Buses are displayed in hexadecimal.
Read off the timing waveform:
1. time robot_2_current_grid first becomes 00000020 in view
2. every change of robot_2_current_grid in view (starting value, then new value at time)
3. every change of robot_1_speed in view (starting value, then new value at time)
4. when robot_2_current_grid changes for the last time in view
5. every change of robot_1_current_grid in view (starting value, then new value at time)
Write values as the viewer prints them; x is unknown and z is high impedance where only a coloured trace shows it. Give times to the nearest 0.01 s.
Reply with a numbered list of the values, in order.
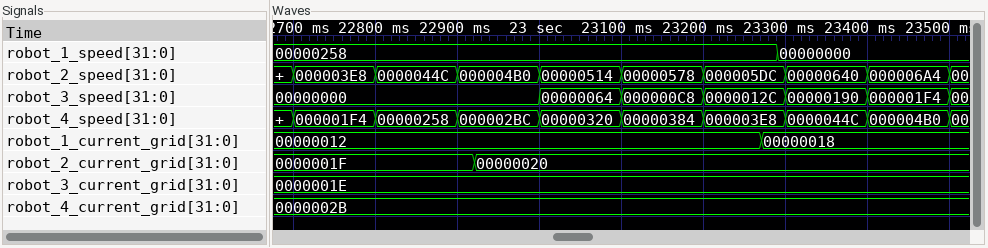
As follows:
1. 22.92 s
2. 0000001F, 00000020 at 22.92 s
3. 00000258, 00000000 at 23.29 s
4. 22.92 s
5. 00000012, 00000018 at 23.27 s
